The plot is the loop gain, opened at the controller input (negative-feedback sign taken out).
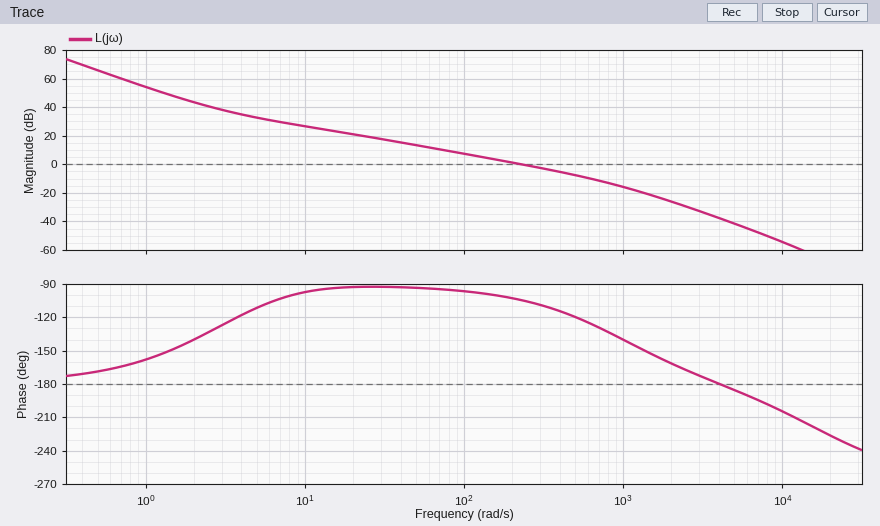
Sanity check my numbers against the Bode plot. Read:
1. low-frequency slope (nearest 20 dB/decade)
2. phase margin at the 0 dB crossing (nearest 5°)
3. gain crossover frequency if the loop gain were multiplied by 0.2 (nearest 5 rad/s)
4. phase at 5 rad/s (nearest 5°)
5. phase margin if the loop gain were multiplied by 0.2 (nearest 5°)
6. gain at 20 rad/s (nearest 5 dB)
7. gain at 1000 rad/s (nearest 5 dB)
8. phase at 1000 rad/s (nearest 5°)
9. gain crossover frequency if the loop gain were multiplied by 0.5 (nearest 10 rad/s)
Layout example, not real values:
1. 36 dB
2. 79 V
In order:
1. -40 dB/decade
2. 75°
3. 45 rad/s
4. -110°
5. 85°
6. 20 dB
7. -15 dB
8. -140°
9. 120 rad/s
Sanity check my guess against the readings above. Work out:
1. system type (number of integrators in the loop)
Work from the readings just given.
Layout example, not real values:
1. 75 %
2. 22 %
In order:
1. 2
